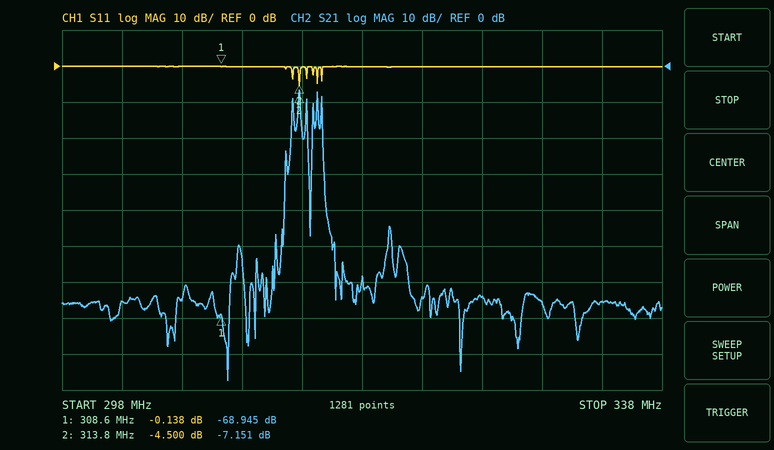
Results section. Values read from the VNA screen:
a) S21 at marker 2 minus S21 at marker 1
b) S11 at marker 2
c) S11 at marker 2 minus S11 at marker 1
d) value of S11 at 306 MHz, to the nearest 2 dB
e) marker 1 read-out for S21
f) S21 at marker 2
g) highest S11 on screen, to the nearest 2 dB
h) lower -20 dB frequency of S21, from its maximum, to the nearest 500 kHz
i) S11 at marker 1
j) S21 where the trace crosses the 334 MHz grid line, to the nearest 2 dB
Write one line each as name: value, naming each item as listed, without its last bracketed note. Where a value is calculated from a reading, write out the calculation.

S21 at marker 2 minus S21 at marker 1: -7.151 − (-68.945) = 61.794 dB
S11 at marker 2: -4.500 dB
S11 at marker 2 minus S11 at marker 1: -4.5 − (-0.138) = -4.362 dB
value of S11 at 306 MHz, to the nearest 2 dB: 0 dB
marker 1 read-out for S21: -68.945 dB
S21 at marker 2: -7.151 dB
highest S11 on screen, to the nearest 2 dB: 0 dB
lower -20 dB frequency of S21, from its maximum, to the nearest 500 kHz: 313.0 MHz
S11 at marker 1: -0.138 dB
S21 where the trace crosses the 334 MHz grid line, to the nearest 2 dB: -66 dB
